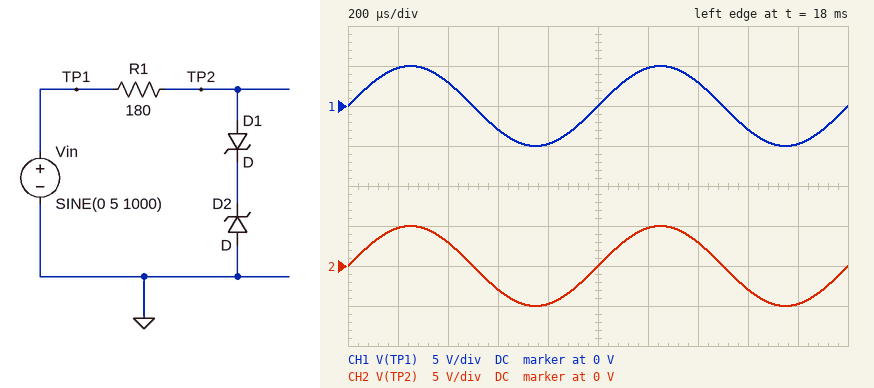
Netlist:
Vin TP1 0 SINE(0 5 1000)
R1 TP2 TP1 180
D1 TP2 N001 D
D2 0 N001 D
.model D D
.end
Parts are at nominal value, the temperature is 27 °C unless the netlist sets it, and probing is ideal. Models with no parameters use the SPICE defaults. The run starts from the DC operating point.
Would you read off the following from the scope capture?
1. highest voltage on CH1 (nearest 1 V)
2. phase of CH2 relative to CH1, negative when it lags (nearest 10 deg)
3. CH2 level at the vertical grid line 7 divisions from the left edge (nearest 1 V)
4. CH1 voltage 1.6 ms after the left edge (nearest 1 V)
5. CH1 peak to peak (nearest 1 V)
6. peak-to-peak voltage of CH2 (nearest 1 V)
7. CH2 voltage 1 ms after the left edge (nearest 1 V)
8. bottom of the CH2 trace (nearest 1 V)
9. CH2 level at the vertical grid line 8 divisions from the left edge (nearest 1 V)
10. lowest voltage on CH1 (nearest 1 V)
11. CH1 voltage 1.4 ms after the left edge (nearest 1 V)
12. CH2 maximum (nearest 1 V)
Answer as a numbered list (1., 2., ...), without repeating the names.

1. 5 V
2. 0 deg
3. 3 V
4. -3 V
5. 10 V
6. 10 V
7. 0 V
8. -5 V
9. -3 V
10. -5 V
11. 3 V
12. 5 V
